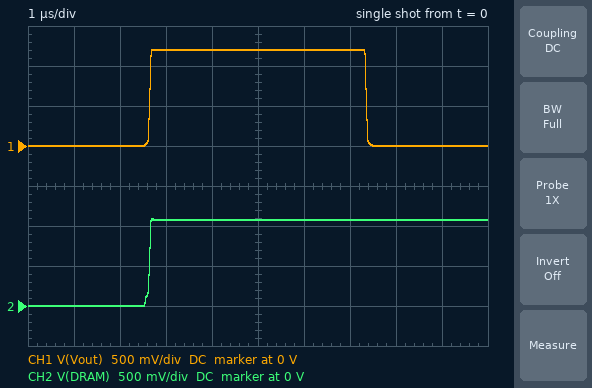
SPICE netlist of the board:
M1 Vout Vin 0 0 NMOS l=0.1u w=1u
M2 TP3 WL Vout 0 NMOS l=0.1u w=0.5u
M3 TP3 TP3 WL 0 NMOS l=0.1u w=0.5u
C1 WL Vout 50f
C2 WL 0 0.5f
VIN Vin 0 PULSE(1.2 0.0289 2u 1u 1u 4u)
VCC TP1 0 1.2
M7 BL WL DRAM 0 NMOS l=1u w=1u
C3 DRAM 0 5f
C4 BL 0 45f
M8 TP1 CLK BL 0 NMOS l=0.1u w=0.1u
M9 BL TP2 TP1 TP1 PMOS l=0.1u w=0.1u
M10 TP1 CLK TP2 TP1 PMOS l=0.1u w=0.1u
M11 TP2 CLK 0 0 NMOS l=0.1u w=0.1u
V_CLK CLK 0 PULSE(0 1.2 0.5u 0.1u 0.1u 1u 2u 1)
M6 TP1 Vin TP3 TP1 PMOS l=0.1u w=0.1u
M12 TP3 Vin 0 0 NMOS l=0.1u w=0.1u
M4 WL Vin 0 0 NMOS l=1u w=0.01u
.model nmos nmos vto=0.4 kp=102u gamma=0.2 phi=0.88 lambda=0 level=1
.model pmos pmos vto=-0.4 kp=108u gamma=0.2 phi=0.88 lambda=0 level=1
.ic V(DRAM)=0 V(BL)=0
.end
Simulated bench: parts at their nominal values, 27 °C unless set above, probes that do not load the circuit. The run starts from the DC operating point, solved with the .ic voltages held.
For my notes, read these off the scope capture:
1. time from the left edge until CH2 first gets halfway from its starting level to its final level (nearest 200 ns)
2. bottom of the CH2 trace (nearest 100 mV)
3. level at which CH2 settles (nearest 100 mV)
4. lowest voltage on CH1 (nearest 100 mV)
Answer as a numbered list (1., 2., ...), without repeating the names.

1. 2.6 µs
2. 0 V
3. 1.1 V
4. 0 V
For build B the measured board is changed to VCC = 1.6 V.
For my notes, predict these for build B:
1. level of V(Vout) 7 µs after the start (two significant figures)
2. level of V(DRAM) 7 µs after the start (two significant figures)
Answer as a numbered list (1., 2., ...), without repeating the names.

1. 1.6 V
2. 1.4 V
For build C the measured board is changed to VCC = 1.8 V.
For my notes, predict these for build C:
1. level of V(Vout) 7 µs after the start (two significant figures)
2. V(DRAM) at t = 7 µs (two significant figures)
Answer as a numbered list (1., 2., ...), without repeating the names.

1. 1.8 V
2. 1.6 V
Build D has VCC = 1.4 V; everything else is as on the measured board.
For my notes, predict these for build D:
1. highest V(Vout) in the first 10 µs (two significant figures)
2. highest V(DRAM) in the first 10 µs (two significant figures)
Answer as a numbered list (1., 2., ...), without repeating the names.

1. 1.4 V
2. 1.3 V
